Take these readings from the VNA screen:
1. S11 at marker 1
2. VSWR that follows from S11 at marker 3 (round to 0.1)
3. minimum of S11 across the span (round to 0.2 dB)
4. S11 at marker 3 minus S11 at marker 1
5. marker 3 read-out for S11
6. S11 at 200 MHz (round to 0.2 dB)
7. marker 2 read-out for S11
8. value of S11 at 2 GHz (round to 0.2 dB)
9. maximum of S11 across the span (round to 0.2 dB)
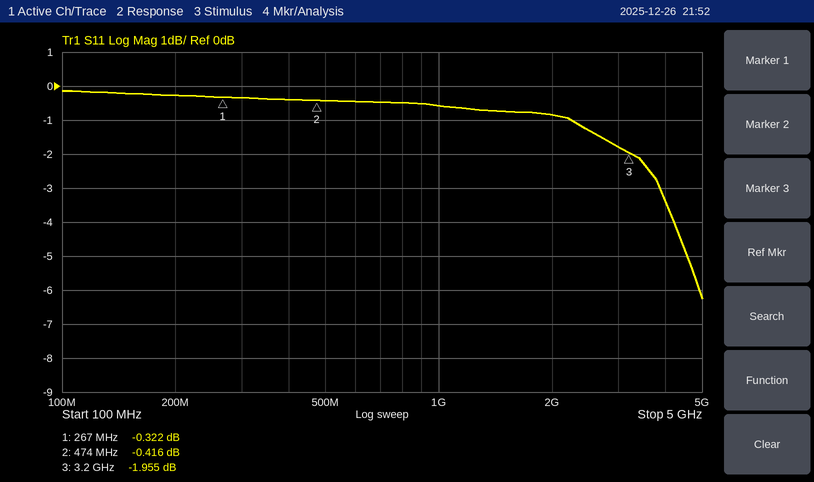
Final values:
-0.322 dB
8.9
-6.2 dB
-1.633 dB
-1.955 dB
-0.2 dB
-0.416 dB
-0.8 dB
-0.2 dB
